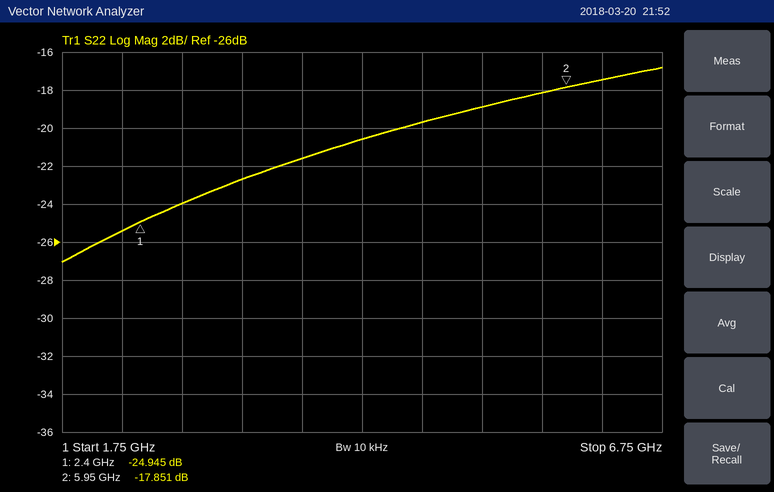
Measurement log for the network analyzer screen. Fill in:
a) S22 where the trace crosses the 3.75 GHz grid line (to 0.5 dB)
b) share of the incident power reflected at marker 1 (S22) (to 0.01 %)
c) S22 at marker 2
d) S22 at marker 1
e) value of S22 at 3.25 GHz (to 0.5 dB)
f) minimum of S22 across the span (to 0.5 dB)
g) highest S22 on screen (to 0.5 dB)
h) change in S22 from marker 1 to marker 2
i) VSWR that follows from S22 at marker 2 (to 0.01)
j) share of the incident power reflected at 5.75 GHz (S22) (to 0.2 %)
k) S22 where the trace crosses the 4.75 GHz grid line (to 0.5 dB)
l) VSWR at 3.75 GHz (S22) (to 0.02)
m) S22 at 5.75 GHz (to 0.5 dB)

-21.5 dB
0.32 %
-17.851 dB
-24.945 dB
-22.5 dB
-27.0 dB
-17.0 dB
7.094 dB
1.29
1.6 %
-19.5 dB
1.18
-18.0 dB
